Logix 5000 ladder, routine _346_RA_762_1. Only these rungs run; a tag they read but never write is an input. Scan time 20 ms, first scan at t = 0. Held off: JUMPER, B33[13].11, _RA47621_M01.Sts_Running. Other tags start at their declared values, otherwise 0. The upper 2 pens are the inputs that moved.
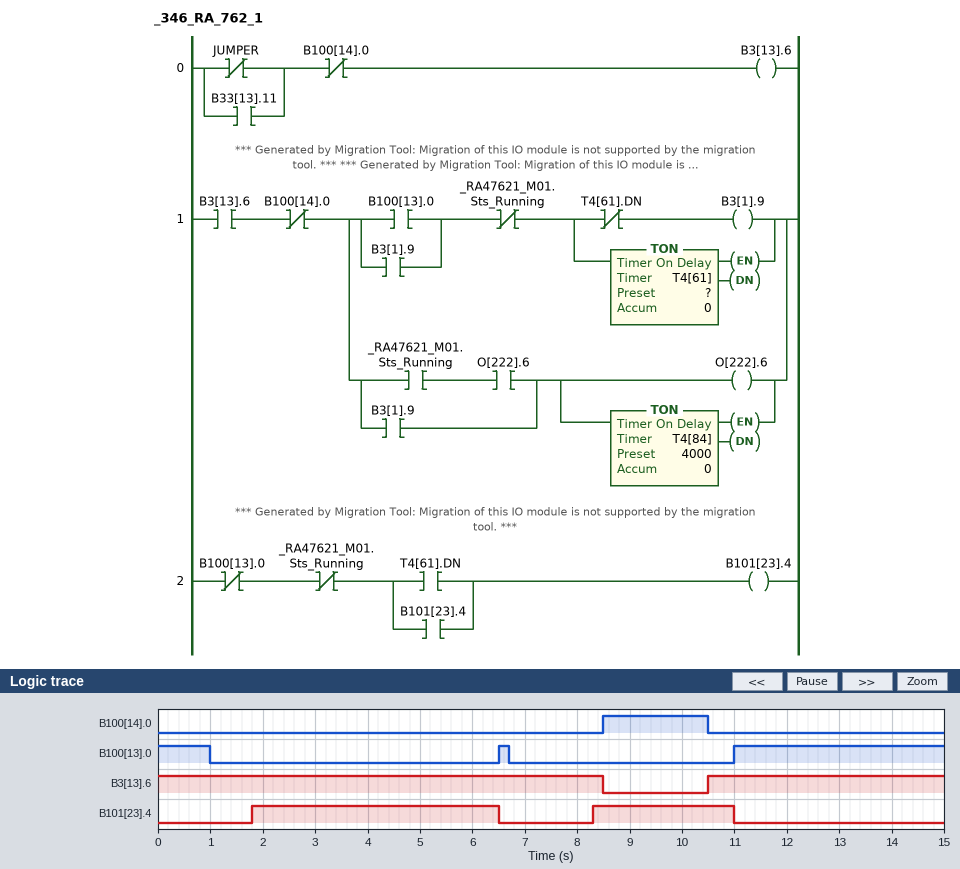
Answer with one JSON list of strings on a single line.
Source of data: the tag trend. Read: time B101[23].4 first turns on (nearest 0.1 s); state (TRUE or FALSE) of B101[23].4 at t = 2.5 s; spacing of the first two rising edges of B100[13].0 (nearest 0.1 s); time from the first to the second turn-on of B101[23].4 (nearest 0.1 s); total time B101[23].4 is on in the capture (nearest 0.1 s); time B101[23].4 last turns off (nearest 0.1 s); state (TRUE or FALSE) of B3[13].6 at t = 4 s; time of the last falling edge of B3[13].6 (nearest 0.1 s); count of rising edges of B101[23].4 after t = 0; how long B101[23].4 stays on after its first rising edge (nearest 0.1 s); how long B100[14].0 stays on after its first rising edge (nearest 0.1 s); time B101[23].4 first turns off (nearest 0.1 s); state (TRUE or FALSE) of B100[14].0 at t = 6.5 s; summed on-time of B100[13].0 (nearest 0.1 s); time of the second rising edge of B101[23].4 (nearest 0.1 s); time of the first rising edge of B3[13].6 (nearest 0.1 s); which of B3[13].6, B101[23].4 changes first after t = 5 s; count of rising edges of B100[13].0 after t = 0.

["1.8 s", "TRUE", "4.5 s", "6.5 s", "7.4 s", "11.0 s", "TRUE", "8.5 s", "2", "4.7 s", "2.0 s", "6.5 s", "FALSE", "5.2 s", "8.3 s", "10.5 s", "B101[23].4", "2"]
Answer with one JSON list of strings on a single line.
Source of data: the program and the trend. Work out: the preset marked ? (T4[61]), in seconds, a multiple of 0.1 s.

["1.8 s"]
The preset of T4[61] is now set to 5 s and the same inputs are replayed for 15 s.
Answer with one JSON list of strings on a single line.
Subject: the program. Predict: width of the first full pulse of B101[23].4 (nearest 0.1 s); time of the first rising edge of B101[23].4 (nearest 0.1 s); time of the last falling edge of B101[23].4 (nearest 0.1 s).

["1.5 s", "5.0 s", "6.5 s"]
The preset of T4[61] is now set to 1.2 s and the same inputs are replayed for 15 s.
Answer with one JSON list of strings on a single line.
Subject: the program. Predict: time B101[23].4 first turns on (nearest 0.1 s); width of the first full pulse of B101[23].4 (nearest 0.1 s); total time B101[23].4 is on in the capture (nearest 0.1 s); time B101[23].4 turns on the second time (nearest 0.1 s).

["1.2 s", "5.3 s", "8.6 s", "7.7 s"]
